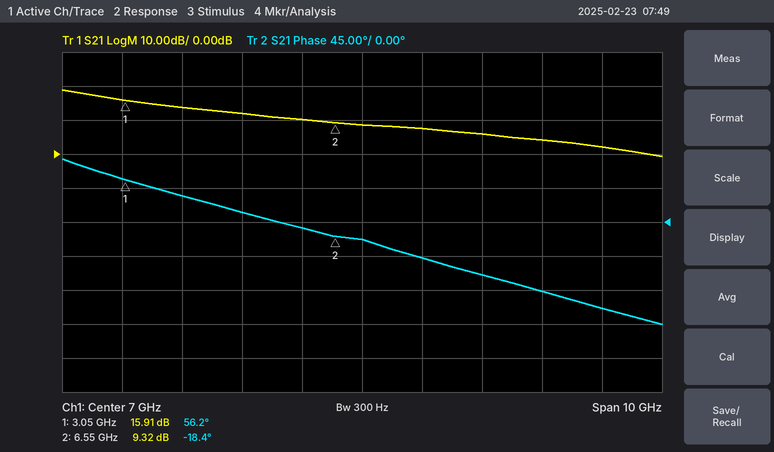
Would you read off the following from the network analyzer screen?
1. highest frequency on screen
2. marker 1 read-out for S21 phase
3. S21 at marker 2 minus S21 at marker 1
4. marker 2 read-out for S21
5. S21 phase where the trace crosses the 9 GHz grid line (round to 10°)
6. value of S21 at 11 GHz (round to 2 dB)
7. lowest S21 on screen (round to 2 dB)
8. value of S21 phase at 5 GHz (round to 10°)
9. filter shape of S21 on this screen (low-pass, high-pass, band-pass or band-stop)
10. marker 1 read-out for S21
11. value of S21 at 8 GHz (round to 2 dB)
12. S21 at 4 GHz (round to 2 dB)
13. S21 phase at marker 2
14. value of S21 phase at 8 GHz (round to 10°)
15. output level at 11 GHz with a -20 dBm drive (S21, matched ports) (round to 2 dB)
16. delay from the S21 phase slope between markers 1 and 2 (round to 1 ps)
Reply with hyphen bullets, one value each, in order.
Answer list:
- 12 GHz
- 56.2°
- -6.59 dB
- 9.32 dB
- -70°
- 2 dB
- 0 dB
- 10°
- low-pass
- 15.91 dB
- 8 dB
- 14 dB
- -18.4°
- -50°
- -18 dBm
- 59 ps
